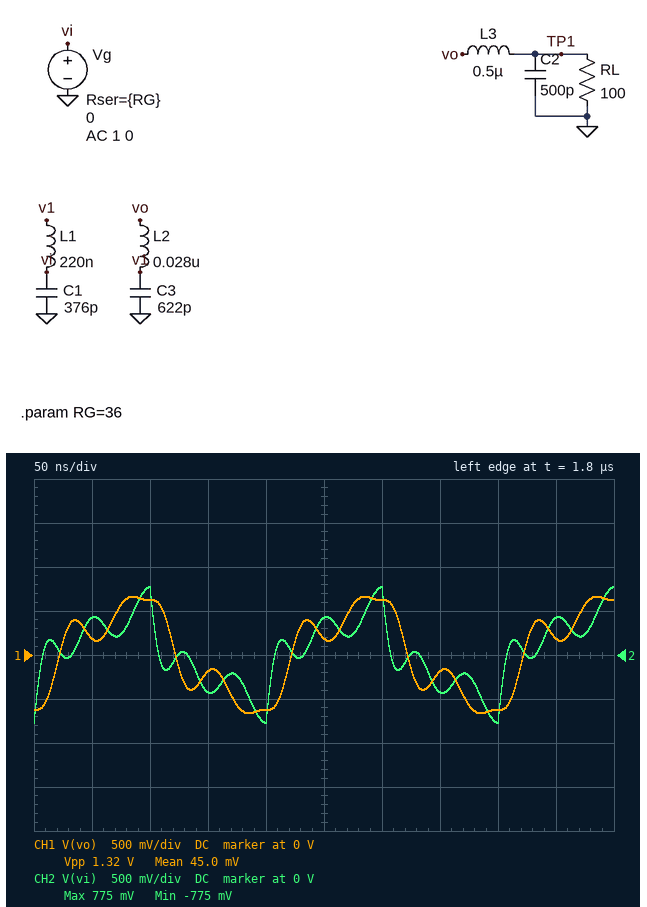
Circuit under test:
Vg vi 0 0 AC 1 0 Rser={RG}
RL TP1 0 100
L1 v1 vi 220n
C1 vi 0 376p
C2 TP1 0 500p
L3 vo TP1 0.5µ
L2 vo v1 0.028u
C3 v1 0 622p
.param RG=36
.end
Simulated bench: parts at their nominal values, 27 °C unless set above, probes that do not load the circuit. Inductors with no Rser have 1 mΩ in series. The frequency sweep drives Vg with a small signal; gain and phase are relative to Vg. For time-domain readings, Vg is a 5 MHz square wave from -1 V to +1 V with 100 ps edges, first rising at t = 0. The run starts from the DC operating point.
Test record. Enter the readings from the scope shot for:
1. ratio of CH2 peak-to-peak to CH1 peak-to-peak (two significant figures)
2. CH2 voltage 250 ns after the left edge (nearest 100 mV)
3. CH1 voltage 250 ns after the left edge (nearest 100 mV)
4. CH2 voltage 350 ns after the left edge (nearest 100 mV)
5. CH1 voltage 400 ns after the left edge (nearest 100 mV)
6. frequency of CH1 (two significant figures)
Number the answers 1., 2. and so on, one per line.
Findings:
1. 1.2
2. 400 mV
3. 200 mV
4. -400 mV
5. -600 mV
6. 5.0 MHz
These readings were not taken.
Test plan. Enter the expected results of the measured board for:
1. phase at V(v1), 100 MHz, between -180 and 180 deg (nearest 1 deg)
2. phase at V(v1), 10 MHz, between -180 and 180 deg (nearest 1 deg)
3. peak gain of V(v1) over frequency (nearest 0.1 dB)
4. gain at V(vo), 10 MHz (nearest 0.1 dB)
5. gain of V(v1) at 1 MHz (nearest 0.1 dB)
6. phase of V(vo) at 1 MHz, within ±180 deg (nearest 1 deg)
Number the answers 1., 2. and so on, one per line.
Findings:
1. 97 deg
2. -32 deg
3. -1.4 dB
4. -12.1 dB
5. -2.9 dB
6. -14 deg
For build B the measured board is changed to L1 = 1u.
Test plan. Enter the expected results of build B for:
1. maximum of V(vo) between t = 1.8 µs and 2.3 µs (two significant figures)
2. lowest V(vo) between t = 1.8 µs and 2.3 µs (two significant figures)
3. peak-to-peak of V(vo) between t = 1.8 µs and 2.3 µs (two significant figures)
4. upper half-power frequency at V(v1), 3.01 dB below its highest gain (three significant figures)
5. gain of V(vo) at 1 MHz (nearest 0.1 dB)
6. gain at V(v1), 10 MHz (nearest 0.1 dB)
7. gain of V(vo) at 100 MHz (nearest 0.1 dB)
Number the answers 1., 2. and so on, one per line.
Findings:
1. 800 mV
2. -800 mV
3. 1.6 V
4. 14.9 MHz
5. -2.8 dB
6. -16.3 dB
7. -66.8 dB
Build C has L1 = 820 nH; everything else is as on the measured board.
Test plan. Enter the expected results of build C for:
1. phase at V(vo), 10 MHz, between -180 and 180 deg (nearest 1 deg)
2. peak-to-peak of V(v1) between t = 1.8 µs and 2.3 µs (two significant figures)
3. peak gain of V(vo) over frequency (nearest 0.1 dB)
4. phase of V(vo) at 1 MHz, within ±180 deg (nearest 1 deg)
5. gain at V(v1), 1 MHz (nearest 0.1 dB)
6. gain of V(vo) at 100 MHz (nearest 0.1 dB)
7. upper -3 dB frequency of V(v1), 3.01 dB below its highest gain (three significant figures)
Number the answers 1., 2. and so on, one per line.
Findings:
1. -95 deg
2. 1.7 V
3. -1.0 dB
4. -16 deg
5. -2.8 dB
6. -65.0 dB
7. 15.2 MHz
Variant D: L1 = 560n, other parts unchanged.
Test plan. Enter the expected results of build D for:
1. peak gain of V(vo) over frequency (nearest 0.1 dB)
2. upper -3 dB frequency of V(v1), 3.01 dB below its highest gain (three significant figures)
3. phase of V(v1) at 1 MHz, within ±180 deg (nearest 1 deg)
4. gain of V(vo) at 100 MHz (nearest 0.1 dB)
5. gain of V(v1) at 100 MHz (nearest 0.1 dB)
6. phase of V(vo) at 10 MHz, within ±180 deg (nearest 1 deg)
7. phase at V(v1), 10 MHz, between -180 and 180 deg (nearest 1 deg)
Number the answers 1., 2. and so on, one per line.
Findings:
1. 0.4 dB
2. 16.4 MHz
3. -15 deg
4. -61.7 dB
5. -61.2 dB
6. -77 deg
7. -68 deg
